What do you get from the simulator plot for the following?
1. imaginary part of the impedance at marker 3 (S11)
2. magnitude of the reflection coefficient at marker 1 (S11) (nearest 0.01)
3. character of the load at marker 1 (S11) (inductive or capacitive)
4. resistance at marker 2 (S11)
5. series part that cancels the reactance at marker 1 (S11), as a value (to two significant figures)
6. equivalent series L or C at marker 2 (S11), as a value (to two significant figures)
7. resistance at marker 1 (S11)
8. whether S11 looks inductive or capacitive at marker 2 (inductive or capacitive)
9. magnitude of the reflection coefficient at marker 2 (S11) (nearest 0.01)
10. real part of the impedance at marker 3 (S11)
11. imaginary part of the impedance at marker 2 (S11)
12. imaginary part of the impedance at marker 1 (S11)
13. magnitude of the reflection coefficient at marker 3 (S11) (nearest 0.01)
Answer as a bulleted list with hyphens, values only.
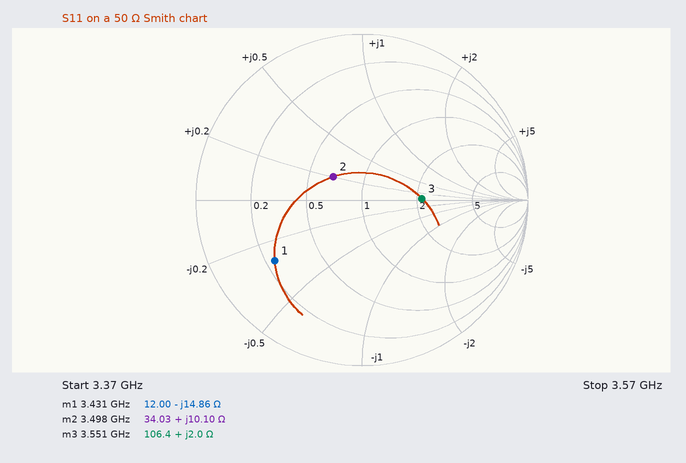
- +2.0 Ω
- 0.64
- capacitive
- 34.03 Ω
- 690 pH
- 460 pH
- 12.00 Ω
- inductive
- 0.22
- 106.4 Ω
- +10.10 Ω
- -14.86 Ω
- 0.36
